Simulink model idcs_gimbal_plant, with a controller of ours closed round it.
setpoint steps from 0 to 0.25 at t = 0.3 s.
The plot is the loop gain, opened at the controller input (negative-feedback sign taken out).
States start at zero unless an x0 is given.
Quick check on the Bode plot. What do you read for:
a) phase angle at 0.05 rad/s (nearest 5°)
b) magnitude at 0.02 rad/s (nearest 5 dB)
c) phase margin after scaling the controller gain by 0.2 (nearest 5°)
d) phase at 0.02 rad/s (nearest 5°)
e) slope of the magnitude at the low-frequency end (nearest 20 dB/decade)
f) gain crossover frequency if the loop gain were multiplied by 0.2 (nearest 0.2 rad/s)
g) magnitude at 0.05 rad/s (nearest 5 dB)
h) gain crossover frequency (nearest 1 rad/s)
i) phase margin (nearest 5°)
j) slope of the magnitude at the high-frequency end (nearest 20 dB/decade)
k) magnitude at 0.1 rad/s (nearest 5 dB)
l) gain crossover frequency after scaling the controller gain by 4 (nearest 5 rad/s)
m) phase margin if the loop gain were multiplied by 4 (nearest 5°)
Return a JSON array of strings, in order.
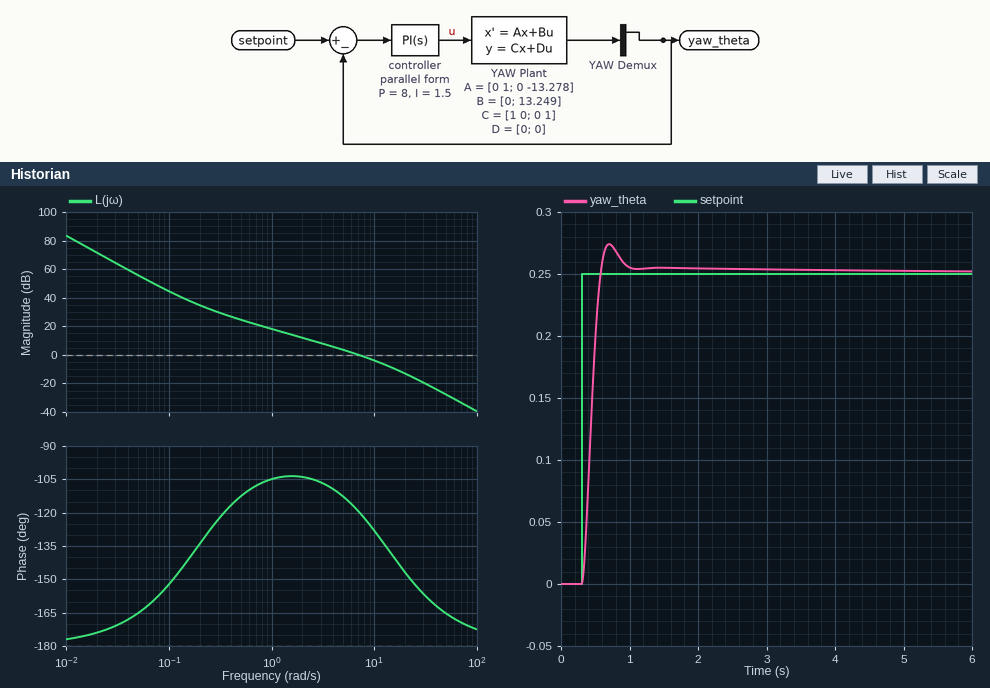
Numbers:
["-165°", "70 dB", "75°", "-175°", "-40 dB/decade", "1.6 rad/s", "55 dB", "7 rad/s", "60°", "-40 dB/decade", "45 dB", "20 rad/s", "35°"]
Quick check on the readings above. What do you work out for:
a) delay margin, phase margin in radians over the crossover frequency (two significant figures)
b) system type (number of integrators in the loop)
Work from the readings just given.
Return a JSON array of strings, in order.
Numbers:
["0.15 s", "2"]
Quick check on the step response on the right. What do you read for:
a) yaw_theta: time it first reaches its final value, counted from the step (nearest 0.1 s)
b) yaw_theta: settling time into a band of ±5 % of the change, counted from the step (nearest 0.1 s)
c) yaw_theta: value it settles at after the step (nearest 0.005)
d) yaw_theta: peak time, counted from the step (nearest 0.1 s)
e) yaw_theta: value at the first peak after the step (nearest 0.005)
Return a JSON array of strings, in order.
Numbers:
["0.3 s", "0.6 s", "0.250", "0.4 s", "0.275"]
